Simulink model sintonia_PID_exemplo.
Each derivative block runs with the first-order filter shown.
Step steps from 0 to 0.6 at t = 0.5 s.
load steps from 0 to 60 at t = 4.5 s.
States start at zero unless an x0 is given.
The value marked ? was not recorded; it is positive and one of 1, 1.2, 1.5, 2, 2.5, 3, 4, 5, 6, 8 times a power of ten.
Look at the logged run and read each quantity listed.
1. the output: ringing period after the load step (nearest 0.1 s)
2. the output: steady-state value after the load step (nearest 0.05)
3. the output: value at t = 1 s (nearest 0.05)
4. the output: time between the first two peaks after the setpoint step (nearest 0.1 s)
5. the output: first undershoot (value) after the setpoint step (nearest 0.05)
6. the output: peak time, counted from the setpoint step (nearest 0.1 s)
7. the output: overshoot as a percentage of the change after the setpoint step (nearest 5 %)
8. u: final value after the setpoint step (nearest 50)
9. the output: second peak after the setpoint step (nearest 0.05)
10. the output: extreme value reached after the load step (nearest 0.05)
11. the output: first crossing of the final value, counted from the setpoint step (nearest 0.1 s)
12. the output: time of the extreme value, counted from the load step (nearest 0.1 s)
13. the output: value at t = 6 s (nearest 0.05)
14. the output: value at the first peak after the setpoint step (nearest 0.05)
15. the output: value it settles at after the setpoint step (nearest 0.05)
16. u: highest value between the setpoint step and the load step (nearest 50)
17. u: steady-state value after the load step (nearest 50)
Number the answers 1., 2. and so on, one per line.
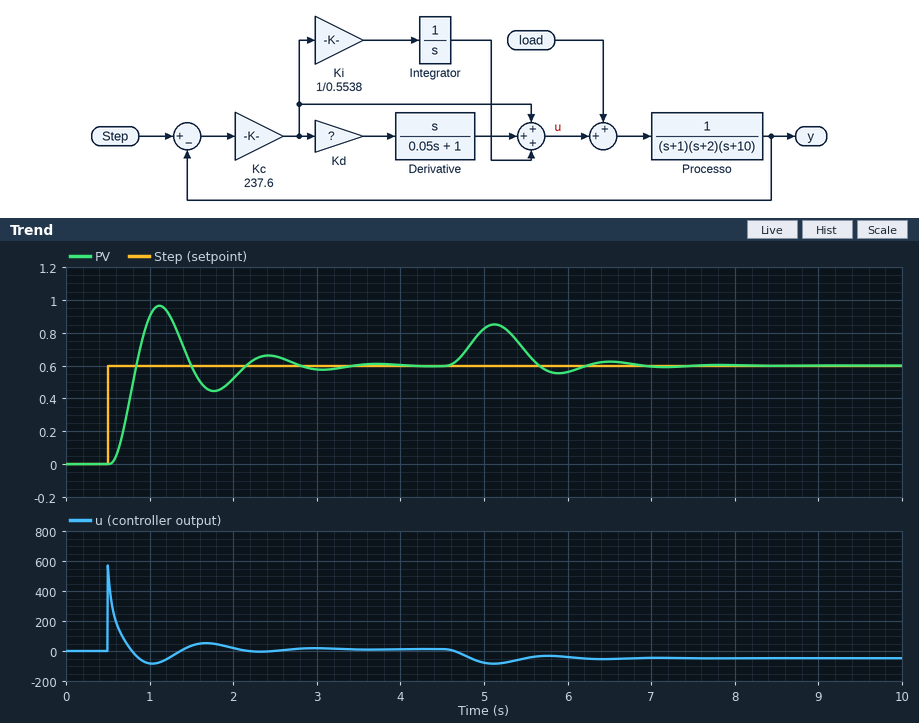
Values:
1. 1.4 s
2. 0.60
3. 0.90
4. 1.3 s
5. 0.45
6. 0.6 s
7. 60 %
8. 0
9. 0.65
10. 0.85
11. 0.3 s
12. 0.6 s
13. 0.55
14. 0.95
15. 0.60
16. 550
17. -50
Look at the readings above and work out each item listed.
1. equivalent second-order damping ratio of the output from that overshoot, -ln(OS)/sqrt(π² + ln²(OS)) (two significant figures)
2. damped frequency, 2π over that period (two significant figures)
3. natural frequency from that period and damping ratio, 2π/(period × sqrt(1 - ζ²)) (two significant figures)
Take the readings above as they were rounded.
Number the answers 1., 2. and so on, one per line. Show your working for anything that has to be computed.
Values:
1. ln(0.6) = -0.511; 0.511 / sqrt(9.870 + 0.261) = 0.16
2. 2π / 1.3 = 4.8 rad/s
3. 2π / (1.3 × sqrt(1 - 0.16²)) = 4.9 rad/s
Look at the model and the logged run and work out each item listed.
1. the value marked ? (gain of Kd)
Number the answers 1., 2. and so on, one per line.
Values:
1. 0.15
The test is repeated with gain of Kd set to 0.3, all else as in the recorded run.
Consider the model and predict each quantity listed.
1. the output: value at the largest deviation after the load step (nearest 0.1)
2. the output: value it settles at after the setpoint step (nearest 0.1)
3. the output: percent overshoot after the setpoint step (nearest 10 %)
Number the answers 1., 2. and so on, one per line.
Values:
1. 0.8
2. 0.6
3. 40 %
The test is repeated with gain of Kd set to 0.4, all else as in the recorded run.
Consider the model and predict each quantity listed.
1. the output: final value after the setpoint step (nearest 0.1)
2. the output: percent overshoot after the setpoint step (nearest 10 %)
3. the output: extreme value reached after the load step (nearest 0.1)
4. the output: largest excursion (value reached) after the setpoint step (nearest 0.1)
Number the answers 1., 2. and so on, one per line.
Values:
1. 0.6
2. 40 %
3. 0.8
4. 0.8
